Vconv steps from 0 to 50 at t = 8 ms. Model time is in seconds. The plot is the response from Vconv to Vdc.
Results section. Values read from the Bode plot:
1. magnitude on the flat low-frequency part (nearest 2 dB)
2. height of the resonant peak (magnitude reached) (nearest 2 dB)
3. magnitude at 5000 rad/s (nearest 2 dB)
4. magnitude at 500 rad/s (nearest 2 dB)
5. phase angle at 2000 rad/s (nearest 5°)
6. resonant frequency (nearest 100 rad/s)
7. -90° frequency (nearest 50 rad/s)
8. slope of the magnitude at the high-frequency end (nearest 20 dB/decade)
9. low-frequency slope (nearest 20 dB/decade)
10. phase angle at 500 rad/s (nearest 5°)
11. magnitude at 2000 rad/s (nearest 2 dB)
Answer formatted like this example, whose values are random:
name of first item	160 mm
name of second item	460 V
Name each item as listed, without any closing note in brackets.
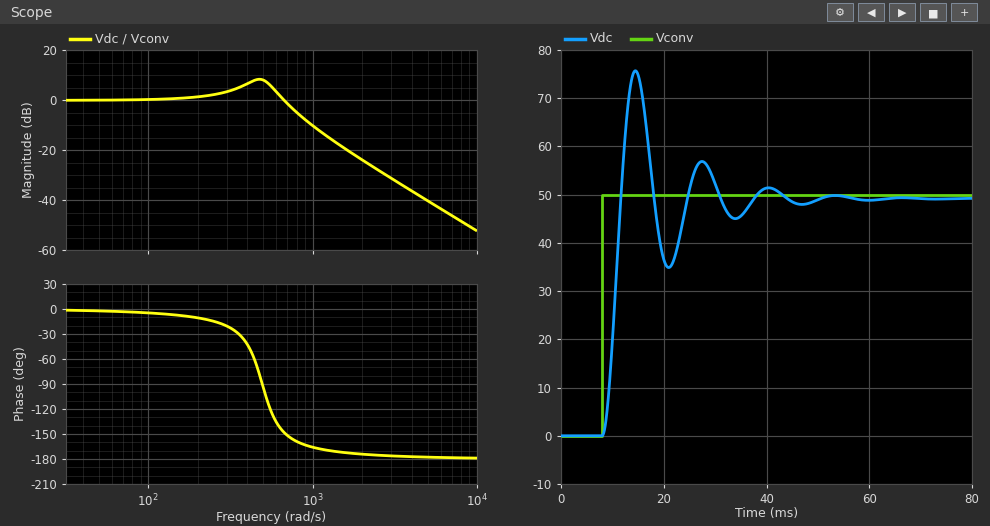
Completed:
magnitude on the flat low-frequency part	0 dB
height of the resonant peak (magnitude reached)	8 dB
magnitude at 5000 rad/s	-40 dB
magnitude at 500 rad/s	8 dB
phase angle at 2000 rad/s	-175°
resonant frequency	500 rad/s
-90° frequency	500 rad/s
slope of the magnitude at the high-frequency end	-40 dB/decade
low-frequency slope	0 dB/decade
phase angle at 500 rad/s	-95°
magnitude at 2000 rad/s	-24 dB
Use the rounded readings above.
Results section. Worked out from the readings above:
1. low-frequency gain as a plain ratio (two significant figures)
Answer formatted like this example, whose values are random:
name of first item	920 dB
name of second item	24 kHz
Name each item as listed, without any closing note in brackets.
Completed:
low-frequency gain as a plain ratio	1.0
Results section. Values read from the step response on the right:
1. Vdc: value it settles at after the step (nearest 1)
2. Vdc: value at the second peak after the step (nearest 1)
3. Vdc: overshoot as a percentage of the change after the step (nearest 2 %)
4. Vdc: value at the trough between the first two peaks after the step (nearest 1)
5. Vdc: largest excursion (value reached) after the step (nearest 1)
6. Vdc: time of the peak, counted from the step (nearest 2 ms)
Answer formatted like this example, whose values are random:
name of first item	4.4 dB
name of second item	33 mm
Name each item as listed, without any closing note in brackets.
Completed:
Vdc: value it settles at after the step	49
Vdc: value at the second peak after the step	57
Vdc: overshoot as a percentage of the change after the step	54 %
Vdc: value at the trough between the first two peaks after the step	35
Vdc: largest excursion (value reached) after the step	76
Vdc: time of the peak, counted from the step	6 ms
